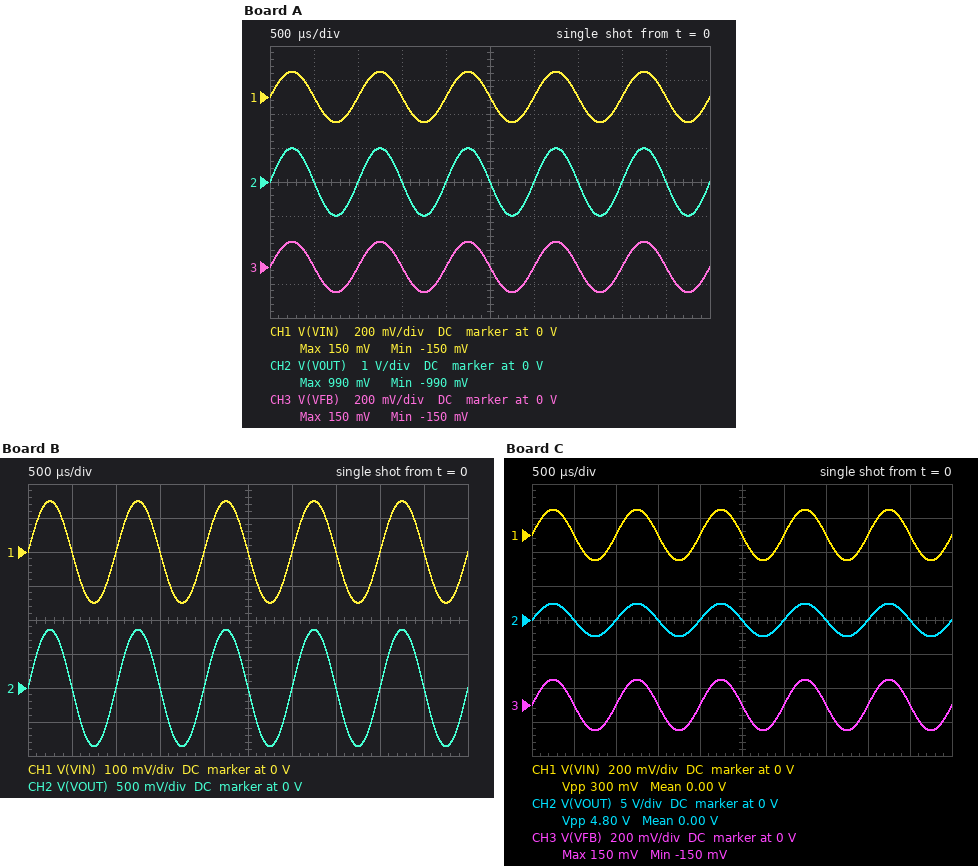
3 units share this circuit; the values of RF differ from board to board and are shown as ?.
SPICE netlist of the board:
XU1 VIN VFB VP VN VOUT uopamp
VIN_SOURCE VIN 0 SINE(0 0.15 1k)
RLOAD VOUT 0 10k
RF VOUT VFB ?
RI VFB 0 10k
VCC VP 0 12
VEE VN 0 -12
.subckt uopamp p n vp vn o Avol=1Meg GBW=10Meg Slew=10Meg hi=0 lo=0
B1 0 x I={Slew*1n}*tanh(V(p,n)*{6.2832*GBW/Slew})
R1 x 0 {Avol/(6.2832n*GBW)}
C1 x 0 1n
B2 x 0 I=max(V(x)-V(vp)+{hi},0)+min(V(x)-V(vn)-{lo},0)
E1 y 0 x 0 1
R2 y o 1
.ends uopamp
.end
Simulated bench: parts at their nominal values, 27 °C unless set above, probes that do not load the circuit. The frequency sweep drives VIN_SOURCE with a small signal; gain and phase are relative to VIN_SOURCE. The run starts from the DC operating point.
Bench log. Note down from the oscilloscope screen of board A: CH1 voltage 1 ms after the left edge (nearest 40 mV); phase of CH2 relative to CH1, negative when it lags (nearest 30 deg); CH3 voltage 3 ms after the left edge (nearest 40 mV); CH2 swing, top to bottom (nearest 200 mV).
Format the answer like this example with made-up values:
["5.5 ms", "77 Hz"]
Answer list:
["0 V", "0 deg", "0 V", "2.0 V"]
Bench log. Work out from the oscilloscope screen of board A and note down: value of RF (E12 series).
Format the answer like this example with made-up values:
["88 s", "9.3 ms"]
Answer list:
["56 kΩ"]
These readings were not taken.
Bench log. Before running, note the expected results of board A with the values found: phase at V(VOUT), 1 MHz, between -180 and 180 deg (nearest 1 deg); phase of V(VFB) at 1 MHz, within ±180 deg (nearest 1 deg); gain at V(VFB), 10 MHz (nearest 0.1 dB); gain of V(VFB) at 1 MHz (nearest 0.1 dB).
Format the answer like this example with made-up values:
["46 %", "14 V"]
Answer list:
["-33 deg", "-33 deg", "-16.5 dB", "-1.6 dB"]
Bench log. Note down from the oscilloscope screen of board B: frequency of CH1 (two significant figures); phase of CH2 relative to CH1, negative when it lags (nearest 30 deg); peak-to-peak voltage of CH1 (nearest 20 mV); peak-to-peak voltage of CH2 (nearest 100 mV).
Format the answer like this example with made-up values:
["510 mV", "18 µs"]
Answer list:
["1.0 kHz", "0 deg", "300 mV", "1.7 V"]
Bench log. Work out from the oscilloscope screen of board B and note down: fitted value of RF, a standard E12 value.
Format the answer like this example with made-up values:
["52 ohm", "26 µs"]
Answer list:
["47 kΩ"]
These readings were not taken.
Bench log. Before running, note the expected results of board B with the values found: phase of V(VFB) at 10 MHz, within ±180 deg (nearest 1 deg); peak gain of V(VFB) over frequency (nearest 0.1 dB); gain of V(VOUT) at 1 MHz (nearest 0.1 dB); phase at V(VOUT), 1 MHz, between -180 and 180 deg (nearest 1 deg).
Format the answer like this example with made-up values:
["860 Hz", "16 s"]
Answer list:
["-80 deg", "0 dB", "13.9 dB", "-30 deg"]
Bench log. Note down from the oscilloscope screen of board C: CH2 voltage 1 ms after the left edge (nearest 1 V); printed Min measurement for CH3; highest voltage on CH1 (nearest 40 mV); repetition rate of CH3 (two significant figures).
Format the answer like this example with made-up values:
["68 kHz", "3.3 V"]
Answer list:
["0 V", "-150 mV", "160 mV", "1.0 kHz"]
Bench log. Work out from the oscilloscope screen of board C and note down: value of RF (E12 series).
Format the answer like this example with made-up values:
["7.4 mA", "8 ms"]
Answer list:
["150 kΩ"]
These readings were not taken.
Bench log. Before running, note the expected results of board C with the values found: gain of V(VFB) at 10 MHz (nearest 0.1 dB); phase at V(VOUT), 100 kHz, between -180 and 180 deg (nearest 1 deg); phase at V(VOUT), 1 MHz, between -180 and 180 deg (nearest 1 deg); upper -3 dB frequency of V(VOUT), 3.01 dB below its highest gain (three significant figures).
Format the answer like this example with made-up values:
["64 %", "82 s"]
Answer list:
["-24.1 dB", "-9 deg", "-58 deg", "625 kHz"]
